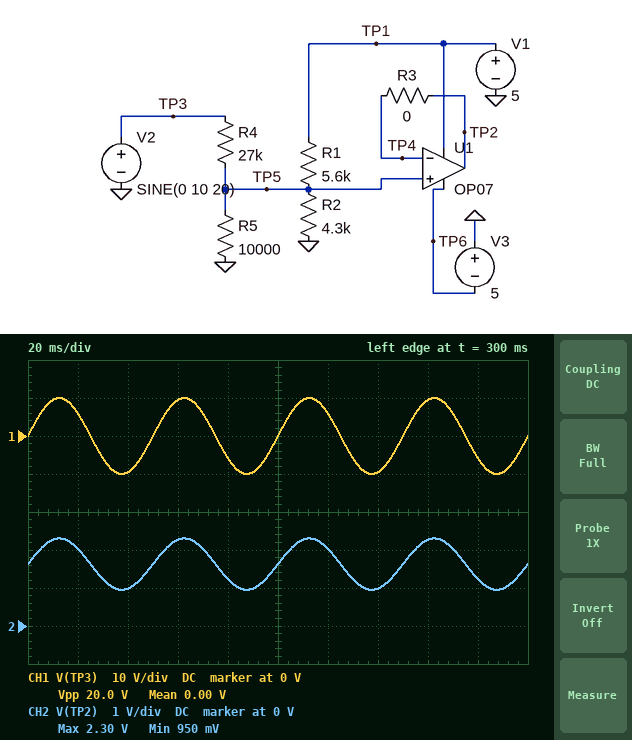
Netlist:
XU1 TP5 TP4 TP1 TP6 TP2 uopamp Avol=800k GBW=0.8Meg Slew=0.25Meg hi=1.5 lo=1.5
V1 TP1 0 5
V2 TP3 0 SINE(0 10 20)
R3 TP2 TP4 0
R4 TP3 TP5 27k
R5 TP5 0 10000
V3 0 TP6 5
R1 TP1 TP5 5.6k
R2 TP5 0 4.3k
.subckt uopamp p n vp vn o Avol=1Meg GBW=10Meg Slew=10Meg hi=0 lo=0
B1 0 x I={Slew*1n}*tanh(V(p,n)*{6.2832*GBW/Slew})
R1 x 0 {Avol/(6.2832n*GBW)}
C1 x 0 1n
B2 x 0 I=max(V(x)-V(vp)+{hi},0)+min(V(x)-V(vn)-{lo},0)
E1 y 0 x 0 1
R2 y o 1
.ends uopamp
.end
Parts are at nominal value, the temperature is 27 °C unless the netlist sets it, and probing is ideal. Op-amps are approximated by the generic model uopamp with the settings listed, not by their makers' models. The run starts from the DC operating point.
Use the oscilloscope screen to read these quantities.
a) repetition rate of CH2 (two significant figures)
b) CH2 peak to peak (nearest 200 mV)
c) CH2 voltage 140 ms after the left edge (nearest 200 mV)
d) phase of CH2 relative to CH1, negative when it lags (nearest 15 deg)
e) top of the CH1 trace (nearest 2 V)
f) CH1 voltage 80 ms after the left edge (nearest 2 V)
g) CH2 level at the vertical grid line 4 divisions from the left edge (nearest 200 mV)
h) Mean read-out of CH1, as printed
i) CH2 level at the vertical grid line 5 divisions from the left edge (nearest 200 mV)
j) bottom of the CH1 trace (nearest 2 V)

20 Hz
1.4 V
1.0 V
0 deg
10 V
-6 V
1.2 V
0.00 V
1.6 V
-10 V
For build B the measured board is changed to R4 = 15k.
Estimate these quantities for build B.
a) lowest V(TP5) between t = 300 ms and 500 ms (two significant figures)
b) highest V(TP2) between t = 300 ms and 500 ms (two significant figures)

390 mV
2.7 V
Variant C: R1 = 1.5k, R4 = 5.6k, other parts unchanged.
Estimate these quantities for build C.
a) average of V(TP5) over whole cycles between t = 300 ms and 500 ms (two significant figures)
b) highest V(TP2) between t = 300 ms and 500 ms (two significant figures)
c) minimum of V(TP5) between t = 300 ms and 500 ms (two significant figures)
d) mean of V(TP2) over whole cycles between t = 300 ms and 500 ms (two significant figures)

2.8 V
3.5 V
1.3 V
2.6 V
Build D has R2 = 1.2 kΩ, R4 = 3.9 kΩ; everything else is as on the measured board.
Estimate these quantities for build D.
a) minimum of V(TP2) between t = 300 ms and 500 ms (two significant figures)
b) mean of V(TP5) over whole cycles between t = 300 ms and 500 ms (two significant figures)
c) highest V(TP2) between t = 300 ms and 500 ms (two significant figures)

-1.2 V
650 mV
2.5 V
